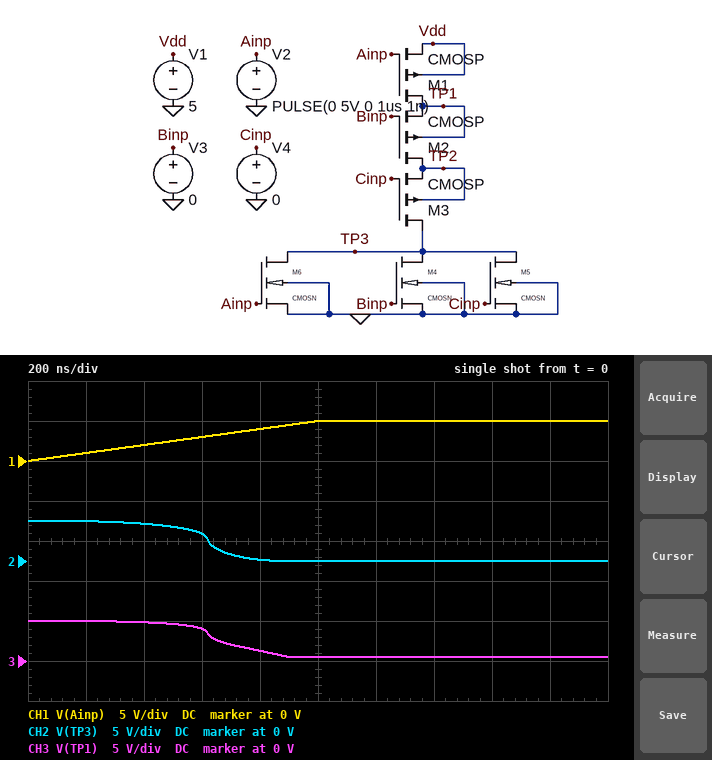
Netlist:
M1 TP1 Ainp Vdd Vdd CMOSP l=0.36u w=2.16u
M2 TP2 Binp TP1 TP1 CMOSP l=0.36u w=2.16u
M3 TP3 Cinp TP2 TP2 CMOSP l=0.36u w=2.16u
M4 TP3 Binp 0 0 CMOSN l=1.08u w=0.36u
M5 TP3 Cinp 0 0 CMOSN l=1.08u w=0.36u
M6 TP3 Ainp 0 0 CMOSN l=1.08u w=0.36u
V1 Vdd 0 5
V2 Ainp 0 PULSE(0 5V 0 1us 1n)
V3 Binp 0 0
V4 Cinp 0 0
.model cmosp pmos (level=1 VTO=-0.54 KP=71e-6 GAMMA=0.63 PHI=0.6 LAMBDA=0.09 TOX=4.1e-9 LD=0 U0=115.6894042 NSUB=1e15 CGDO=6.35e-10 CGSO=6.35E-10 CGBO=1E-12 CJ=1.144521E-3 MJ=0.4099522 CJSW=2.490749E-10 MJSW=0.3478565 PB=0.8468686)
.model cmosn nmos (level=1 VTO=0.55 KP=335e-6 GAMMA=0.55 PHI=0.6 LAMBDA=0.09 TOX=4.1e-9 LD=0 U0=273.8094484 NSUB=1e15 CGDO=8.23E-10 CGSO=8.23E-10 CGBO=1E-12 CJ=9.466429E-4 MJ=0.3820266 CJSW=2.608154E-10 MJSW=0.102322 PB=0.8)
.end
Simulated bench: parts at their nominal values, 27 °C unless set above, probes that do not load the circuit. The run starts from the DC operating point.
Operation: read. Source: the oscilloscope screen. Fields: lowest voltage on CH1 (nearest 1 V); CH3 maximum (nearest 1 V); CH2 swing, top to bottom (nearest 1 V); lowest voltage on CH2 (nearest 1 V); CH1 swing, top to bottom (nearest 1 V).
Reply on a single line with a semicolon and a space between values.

0 V; 5 V; 5 V; 0 V; 5 V
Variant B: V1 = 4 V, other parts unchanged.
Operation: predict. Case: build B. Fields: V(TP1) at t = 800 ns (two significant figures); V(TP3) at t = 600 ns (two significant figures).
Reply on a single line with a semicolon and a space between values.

550 mV; 210 mV
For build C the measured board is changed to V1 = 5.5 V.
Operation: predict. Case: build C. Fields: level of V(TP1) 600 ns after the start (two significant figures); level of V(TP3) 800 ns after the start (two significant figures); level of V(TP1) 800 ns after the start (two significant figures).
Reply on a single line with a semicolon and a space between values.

4.9 V; 700 mV; 2.1 V
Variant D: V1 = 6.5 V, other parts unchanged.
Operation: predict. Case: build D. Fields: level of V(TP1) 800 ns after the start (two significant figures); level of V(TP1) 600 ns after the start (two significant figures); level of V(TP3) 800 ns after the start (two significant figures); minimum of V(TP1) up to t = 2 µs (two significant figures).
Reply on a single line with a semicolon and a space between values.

4.9 V; 6.1 V; 3.9 V; 2.1 V
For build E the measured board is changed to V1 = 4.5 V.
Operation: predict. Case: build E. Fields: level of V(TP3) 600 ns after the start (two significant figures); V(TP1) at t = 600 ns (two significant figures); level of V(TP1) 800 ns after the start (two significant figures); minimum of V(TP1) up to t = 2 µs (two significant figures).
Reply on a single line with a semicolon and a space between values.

1.0 V; 2.1 V; 550 mV; 540 mV
